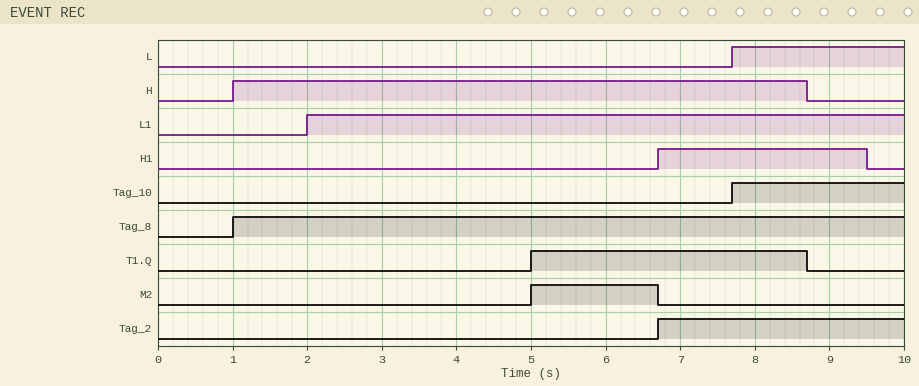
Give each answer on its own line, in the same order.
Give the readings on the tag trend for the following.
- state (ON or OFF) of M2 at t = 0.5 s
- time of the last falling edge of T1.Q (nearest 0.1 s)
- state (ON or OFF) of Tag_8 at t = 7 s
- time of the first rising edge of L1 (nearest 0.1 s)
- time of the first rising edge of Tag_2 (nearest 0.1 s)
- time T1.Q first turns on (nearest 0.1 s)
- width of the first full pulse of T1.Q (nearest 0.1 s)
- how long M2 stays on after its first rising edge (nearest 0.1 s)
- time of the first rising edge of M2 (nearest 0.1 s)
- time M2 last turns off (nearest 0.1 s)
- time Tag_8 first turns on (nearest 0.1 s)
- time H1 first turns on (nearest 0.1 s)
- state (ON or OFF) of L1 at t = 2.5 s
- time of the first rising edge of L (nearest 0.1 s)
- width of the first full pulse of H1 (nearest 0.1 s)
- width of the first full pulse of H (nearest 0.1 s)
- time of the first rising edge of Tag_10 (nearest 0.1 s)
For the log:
OFF
8.7 s
ON
2.0 s
6.7 s
5.0 s
3.7 s
1.7 s
5.0 s
6.7 s
1.0 s
6.7 s
ON
7.7 s
2.8 s
7.7 s
7.7 s
